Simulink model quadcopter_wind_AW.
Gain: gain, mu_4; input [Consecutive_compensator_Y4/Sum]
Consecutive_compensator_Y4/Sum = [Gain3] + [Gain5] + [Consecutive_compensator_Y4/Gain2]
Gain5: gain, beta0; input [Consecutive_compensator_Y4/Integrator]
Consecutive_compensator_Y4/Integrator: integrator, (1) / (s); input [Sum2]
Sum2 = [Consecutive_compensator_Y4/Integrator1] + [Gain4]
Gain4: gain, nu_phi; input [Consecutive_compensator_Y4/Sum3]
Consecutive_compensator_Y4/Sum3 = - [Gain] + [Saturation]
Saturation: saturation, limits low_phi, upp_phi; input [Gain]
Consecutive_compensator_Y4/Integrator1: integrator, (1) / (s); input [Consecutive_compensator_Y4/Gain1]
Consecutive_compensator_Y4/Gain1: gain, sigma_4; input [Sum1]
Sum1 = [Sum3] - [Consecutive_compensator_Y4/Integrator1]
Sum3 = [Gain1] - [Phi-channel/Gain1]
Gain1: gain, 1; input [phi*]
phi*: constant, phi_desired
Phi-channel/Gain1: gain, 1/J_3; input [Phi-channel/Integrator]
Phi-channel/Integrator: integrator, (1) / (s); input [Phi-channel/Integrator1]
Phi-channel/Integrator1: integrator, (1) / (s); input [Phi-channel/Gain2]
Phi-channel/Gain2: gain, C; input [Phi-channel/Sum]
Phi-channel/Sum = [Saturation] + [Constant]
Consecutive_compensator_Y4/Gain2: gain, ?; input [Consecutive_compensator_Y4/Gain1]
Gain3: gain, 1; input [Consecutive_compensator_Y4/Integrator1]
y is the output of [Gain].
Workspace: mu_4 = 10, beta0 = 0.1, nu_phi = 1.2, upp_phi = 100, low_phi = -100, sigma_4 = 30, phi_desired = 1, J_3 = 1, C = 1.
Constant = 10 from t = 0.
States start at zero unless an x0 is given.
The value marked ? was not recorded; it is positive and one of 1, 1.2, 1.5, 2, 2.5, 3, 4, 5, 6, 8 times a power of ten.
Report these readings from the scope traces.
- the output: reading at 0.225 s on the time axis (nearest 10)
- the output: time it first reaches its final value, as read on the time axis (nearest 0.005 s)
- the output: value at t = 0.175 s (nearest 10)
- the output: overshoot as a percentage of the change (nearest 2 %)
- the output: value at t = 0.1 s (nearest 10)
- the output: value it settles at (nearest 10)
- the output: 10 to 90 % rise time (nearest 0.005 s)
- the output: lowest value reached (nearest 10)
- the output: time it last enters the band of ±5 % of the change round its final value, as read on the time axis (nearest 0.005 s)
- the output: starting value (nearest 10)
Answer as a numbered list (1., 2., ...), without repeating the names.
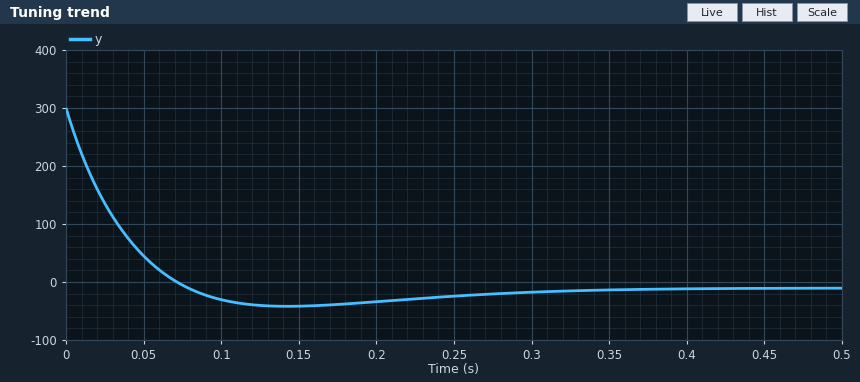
1. -30
2. 0.080 s
3. -40
4. 10 %
5. -30
6. -10
7. 0.055 s
8. -40
9. 0.245 s
10. 300
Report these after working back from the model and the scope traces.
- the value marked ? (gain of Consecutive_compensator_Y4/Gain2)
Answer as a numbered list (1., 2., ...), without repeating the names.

1. 1
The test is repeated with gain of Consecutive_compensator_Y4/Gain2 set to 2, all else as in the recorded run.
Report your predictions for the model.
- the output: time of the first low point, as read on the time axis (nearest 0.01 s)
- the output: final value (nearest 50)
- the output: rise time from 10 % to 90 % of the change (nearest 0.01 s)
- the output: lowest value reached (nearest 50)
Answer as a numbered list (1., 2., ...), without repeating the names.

1. 0.12 s
2. 0
3. 0.05 s
4. -100
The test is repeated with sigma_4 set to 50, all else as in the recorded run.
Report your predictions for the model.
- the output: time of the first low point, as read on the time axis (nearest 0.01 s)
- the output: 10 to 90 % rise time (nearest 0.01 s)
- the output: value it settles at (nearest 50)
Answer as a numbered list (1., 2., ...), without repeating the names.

1. 0.11 s
2. 0.04 s
3. 0
